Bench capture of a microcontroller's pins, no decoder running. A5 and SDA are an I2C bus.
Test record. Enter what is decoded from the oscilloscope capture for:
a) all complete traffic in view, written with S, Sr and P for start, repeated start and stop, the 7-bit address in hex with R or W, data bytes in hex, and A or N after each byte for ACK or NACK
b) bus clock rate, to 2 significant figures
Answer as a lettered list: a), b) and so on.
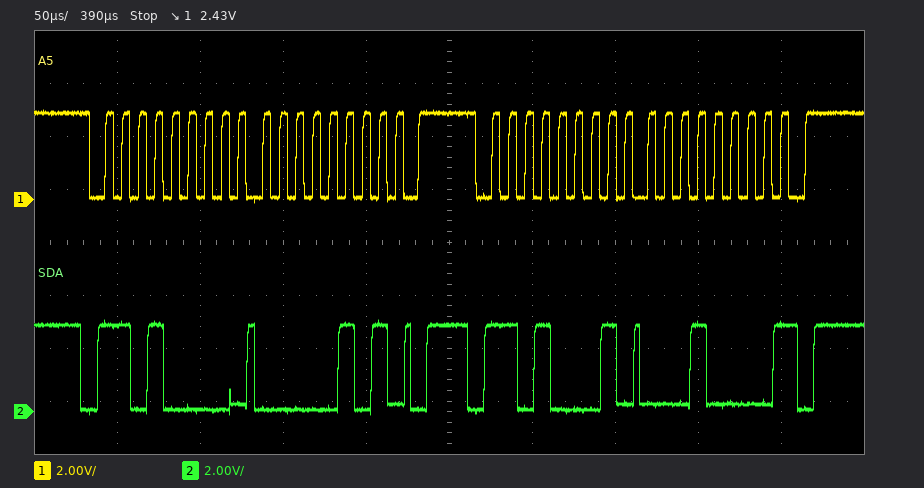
a) S 68W A 05 A P S 68R A 10 N P
b) 100 kHz
